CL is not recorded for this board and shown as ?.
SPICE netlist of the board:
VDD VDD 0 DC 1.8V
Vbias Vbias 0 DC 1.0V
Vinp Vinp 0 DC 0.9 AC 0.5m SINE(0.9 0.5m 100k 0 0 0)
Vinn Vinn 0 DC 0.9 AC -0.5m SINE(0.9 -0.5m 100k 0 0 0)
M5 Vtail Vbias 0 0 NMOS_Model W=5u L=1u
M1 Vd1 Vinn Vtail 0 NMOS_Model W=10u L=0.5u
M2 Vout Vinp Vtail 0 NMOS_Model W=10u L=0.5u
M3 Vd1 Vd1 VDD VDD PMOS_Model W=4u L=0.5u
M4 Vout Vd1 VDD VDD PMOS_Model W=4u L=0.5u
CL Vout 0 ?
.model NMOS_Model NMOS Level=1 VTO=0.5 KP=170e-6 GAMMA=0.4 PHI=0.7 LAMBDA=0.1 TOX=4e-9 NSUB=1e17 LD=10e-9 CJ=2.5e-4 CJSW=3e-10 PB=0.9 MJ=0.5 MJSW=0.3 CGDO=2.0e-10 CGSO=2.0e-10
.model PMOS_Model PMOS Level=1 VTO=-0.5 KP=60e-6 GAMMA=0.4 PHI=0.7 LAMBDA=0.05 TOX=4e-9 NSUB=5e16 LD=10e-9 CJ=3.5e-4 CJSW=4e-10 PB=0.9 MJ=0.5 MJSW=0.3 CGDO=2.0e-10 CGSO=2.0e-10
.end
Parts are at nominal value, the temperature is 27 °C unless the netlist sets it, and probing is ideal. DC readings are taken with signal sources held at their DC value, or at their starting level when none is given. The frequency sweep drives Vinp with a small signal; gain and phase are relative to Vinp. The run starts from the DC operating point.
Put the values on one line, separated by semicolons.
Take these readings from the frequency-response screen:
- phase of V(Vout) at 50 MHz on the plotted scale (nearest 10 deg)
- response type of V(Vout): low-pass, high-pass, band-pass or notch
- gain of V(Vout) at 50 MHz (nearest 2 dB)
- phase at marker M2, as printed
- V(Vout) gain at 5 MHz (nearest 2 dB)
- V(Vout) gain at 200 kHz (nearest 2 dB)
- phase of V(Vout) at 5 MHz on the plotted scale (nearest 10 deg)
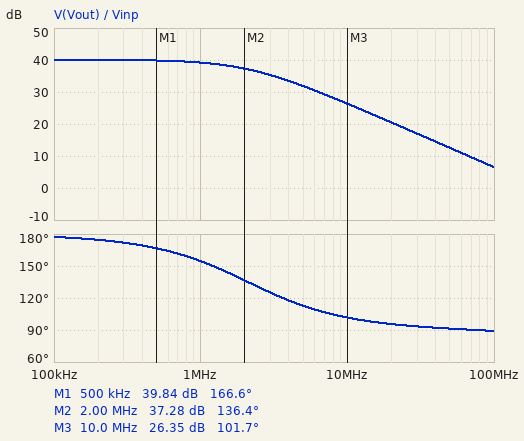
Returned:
90 deg; low-pass; 12 dB; 136.4 deg; 32 dB; 40 dB; 110 deg
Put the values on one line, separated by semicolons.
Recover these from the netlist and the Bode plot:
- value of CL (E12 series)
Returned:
390 fF
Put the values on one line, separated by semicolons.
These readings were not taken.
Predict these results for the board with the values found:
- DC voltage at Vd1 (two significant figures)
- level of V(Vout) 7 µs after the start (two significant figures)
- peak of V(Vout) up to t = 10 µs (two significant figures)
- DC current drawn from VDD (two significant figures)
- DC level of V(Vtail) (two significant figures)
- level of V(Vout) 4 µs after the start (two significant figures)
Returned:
920 mV; 1.0 V; 1.0 V; 74 µA; 210 mV; 860 mV
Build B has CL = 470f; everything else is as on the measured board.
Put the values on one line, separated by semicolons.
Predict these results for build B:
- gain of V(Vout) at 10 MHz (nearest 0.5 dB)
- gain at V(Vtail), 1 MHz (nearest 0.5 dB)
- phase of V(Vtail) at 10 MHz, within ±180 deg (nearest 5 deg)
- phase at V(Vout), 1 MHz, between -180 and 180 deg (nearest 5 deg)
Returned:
25.0 dB; -14.0 dB; 5 deg; 150 deg
